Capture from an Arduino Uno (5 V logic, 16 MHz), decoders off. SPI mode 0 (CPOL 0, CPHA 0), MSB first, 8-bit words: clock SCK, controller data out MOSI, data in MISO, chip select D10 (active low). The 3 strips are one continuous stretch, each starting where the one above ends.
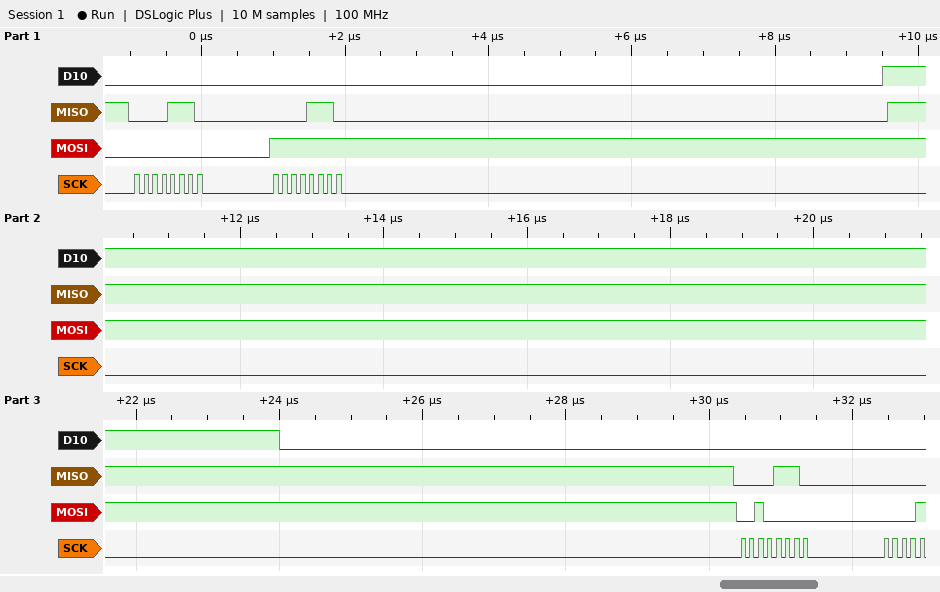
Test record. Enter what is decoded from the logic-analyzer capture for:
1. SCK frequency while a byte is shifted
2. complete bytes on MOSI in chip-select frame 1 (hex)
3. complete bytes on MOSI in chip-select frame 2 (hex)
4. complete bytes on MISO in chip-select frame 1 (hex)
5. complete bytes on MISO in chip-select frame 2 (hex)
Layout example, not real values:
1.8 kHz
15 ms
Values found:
8 MHz
00 FF
20
0E 0E
0E
